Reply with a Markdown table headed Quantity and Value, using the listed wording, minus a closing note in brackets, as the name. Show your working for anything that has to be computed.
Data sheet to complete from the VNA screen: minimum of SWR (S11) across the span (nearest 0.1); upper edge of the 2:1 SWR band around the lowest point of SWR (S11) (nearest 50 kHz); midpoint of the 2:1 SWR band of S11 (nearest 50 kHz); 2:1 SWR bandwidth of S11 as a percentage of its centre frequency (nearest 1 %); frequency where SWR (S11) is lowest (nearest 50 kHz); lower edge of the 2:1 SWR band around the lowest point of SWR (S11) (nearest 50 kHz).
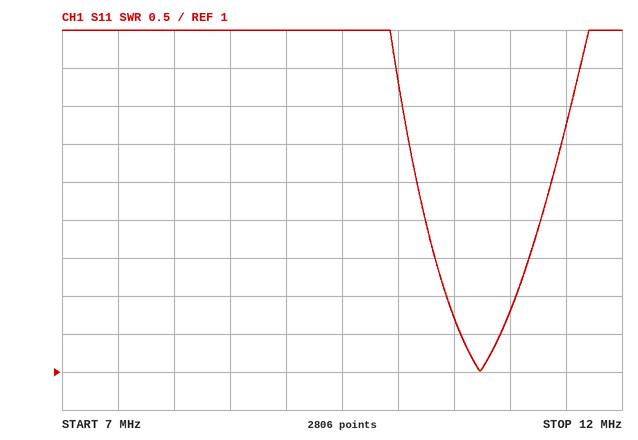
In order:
| Quantity | Value |
|---|---|
| minimum of SWR (S11) across the span | 1.0 |
| upper edge of the 2:1 SWR band around the lowest point of SWR (S11) | 11.05 MHz |
| midpoint of the 2:1 SWR band of S11 | 10.75 MHz |
| 2:1 SWR bandwidth of S11 as a percentage of its centre frequency | 600 kHz / 10.75 MHz ≈ 6 % |
| frequency where SWR (S11) is lowest | 10.75 MHz |
| lower edge of the 2:1 SWR band around the lowest point of SWR (S11) | 10.45 MHz |
